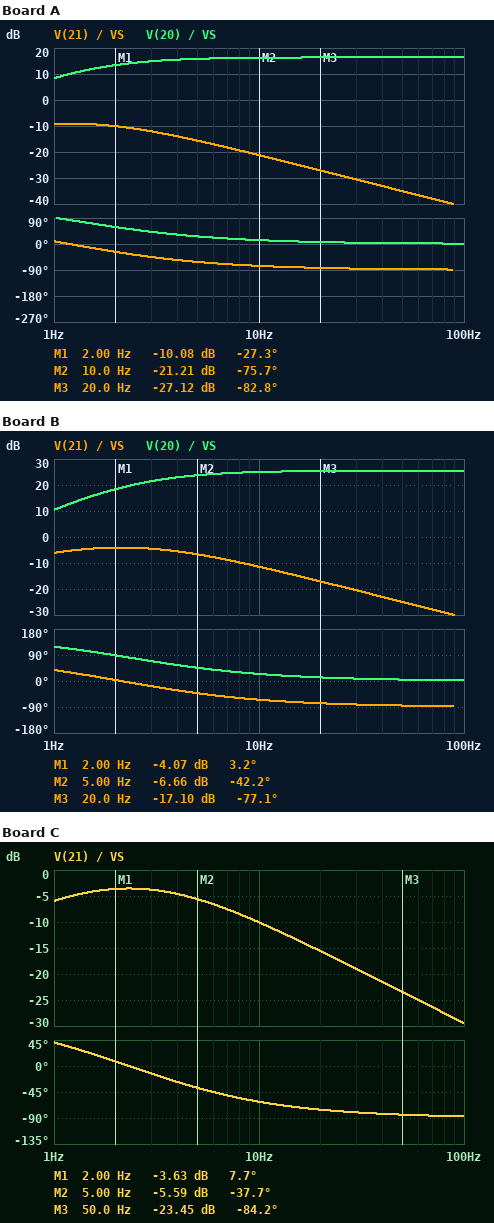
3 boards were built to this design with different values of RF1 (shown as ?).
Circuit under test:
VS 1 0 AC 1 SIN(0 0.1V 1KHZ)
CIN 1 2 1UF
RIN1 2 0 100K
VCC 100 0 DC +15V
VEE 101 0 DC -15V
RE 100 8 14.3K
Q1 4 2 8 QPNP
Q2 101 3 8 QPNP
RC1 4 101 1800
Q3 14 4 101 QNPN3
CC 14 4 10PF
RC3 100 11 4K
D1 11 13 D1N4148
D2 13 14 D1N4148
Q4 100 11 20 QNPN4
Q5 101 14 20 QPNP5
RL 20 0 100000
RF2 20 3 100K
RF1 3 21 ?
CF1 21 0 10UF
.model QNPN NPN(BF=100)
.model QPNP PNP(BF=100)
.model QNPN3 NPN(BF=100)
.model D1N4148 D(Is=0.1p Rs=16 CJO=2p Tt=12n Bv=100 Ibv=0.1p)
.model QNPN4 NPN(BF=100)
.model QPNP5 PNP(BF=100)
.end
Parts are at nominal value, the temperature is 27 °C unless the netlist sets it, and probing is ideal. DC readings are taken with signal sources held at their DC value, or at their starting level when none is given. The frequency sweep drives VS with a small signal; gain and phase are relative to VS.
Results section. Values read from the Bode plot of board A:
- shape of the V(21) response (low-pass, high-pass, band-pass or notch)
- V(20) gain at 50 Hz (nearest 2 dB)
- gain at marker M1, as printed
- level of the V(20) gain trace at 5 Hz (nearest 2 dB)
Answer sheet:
low-pass
16 dB
-10.08 dB
16 dB
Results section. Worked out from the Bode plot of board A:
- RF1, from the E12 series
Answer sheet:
18 kΩ
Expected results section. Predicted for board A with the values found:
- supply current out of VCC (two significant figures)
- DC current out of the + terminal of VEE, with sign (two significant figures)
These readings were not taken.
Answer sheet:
4.6 mA
-4.6 mA
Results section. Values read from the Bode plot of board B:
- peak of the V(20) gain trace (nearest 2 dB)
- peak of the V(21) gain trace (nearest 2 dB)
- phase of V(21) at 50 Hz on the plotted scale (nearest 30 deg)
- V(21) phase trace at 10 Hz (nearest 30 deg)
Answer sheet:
26 dB
-4 dB
-90 deg
-60 deg
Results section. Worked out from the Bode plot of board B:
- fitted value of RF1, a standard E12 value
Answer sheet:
5.6 kΩ
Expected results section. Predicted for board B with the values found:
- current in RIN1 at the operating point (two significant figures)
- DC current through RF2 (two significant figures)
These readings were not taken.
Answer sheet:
4.8 µA
4.7 µA
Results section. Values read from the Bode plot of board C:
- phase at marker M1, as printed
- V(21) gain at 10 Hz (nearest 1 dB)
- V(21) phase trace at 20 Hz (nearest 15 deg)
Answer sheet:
7.7 deg
-10 dB
-75 deg
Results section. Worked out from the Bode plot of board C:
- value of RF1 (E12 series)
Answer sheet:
4.7 kΩ
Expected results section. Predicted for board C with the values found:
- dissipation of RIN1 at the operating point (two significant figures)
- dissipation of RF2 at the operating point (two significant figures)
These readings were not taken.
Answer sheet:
2.3 µW
2.2 µW
